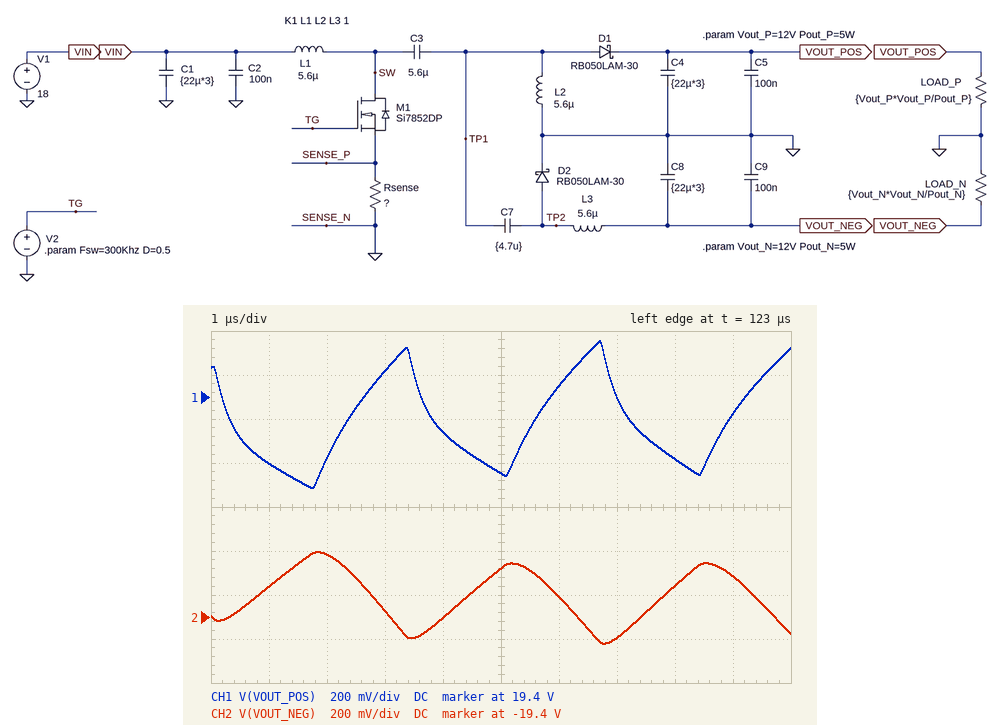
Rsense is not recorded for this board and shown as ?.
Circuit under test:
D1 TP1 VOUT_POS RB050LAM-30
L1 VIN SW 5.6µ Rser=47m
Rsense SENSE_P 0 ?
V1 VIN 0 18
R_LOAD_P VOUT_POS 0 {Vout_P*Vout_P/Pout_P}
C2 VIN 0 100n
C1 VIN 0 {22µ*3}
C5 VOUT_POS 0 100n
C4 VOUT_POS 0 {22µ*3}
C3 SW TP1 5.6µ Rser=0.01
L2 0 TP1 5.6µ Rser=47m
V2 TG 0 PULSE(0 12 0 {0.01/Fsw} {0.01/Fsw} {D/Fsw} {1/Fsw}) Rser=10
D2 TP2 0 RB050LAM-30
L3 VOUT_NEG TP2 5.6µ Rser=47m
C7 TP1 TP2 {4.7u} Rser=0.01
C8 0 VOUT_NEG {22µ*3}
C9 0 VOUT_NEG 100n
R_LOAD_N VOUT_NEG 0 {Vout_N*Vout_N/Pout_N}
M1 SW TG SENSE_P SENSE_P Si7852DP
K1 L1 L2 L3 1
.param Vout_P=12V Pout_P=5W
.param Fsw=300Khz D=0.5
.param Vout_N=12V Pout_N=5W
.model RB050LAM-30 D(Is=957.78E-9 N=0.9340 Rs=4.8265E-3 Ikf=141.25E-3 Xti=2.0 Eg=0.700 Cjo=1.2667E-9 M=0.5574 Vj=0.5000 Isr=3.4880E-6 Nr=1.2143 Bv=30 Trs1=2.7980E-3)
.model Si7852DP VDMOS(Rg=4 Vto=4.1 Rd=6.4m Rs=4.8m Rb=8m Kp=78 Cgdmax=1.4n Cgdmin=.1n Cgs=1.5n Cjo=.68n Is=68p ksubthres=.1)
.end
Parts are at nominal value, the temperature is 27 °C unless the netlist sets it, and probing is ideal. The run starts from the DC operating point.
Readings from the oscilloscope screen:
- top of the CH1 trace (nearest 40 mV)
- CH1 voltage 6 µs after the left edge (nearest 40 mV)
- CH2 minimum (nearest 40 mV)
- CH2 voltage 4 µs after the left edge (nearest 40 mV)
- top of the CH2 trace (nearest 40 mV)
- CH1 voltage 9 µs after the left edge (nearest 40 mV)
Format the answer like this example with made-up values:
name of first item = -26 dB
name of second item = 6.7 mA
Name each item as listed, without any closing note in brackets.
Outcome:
top of the CH1 trace = 19.64 V
CH1 voltage 6 µs after the left edge = 19.44 V
CH2 minimum = -19.52 V
CH2 voltage 4 µs after the left edge = -19.40 V
top of the CH2 trace = -19.12 V
CH1 voltage 9 µs after the left edge = 19.32 V
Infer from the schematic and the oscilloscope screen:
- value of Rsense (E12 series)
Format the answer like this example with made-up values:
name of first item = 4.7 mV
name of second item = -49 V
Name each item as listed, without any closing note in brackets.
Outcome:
value of Rsense = 0.027 Ω
